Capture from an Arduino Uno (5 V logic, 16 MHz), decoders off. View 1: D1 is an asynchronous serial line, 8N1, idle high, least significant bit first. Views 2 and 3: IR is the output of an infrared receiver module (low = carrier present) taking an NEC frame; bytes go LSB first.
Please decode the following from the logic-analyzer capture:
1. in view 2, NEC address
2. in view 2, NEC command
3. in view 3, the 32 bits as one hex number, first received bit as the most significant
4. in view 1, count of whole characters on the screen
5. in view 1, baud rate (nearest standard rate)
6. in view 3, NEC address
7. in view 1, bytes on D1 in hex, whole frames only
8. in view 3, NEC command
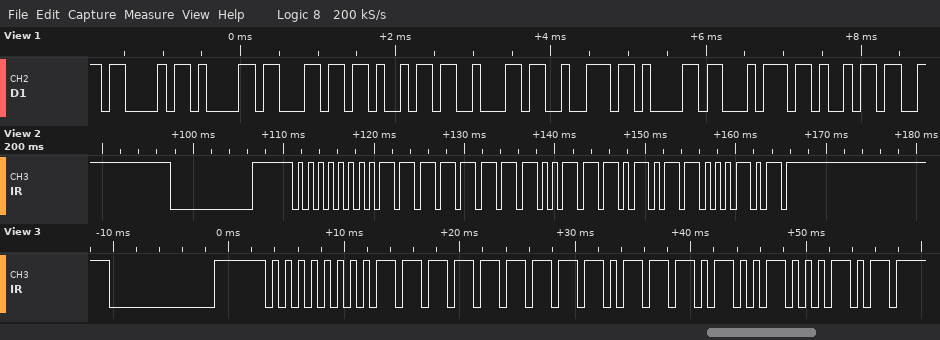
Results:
0x00
0x5C
0x00FFBA45
9
9600 baud
0x00
43 61 6C 69 62 72 61 74 69
0x5D
